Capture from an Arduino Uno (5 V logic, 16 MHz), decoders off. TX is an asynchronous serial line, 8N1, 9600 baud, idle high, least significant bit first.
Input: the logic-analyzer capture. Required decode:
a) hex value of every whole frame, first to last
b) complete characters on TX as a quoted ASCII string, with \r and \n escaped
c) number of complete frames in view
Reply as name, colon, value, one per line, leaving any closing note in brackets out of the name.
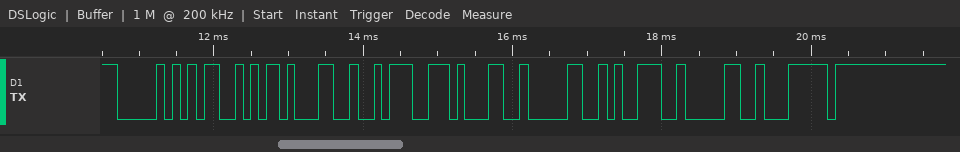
hex value of every whole frame, first to last: 0x50 0x53 0x31 0x3A 0x31 0x30 0x39 0x30 0x7C
complete characters on TX as a quoted ASCII string, with \r and \n escaped: "PS1:1090|"
number of complete frames in view: 9
